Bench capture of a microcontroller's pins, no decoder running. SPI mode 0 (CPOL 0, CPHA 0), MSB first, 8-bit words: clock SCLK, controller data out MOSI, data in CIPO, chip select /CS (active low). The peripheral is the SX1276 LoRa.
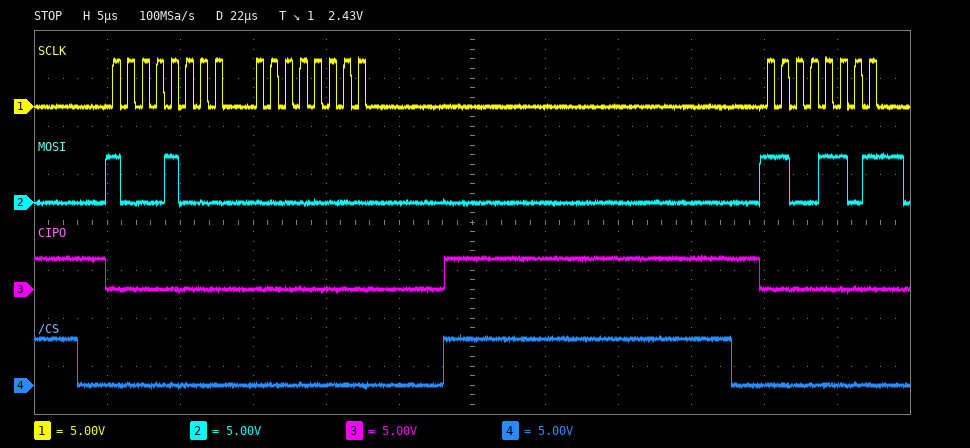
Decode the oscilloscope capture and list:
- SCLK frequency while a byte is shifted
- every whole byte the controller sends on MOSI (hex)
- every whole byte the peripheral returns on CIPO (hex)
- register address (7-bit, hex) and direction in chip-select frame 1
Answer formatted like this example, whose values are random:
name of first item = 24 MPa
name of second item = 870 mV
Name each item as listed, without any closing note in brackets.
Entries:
SCLK frequency while a byte is shifted = 1 MHz
every whole byte the controller sends on MOSI = 88 00 CD
every whole byte the peripheral returns on CIPO = 00 00 00
register address (7-bit, hex) and direction in chip-select frame 1 = 0x08 write
